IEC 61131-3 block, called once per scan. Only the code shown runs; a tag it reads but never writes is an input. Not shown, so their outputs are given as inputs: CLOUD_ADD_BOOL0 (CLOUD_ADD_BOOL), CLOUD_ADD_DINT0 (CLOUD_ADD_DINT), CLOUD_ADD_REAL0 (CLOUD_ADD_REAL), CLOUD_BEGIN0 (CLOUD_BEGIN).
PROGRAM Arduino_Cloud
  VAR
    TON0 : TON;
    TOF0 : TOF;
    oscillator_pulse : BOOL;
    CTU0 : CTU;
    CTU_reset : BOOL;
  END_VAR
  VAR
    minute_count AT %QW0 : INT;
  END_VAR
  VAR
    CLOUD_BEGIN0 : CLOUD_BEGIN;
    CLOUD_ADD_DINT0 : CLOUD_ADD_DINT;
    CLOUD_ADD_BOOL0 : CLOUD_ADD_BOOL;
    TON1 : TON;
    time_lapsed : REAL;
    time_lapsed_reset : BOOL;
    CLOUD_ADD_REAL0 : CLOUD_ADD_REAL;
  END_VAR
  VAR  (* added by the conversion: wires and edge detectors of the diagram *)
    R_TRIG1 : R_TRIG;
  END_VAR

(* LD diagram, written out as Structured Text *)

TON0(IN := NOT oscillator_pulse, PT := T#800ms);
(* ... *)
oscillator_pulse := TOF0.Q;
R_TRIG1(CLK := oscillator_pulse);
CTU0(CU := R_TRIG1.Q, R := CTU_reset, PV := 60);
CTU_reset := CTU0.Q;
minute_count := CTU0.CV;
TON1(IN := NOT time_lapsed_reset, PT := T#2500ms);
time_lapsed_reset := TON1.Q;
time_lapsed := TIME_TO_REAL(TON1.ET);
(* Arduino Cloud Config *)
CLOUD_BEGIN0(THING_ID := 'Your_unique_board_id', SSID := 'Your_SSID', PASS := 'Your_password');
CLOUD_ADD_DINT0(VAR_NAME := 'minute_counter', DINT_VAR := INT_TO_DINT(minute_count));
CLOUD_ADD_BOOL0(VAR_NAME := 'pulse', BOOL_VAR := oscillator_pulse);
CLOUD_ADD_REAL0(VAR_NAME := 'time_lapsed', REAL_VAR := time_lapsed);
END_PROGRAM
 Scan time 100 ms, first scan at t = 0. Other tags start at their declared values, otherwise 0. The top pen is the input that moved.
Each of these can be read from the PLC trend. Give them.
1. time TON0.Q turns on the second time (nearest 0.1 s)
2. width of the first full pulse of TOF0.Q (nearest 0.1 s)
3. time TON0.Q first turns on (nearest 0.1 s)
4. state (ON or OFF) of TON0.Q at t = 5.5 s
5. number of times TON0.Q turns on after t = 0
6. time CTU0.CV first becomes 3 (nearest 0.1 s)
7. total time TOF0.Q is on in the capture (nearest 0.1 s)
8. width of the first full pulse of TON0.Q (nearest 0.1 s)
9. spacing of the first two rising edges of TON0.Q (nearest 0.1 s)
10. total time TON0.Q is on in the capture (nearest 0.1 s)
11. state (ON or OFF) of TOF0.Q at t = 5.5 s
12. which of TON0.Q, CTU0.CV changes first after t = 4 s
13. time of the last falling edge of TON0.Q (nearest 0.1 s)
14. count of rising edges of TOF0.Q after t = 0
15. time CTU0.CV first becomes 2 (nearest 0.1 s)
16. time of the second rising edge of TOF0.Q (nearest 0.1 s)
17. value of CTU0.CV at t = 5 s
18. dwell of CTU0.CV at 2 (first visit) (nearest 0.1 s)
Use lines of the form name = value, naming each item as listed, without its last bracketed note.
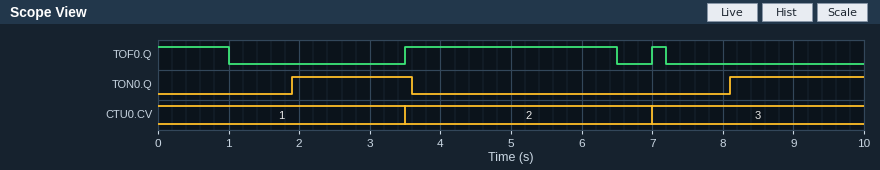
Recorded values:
time TON0.Q turns on the second time = 8.1 s
width of the first full pulse of TOF0.Q = 3.0 s
time TON0.Q first turns on = 1.9 s
state (ON or OFF) of TON0.Q at t = 5.5 s = OFF
number of times TON0.Q turns on after t = 0 = 2
time CTU0.CV first becomes 3 = 7.0 s
total time TOF0.Q is on in the capture = 4.2 s
width of the first full pulse of TON0.Q = 1.7 s
spacing of the first two rising edges of TON0.Q = 6.2 s
total time TON0.Q is on in the capture = 3.6 s
state (ON or OFF) of TOF0.Q at t = 5.5 s = ON
which of TON0.Q, CTU0.CV changes first after t = 4 s = CTU0.CV
time of the last falling edge of TON0.Q = 3.6 s
count of rising edges of TOF0.Q after t = 0 = 2
time CTU0.CV first becomes 2 = 3.5 s
time of the second rising edge of TOF0.Q = 7.0 s
value of CTU0.CV at t = 5 s = 2
dwell of CTU0.CV at 2 (first visit) = 3.5 s
